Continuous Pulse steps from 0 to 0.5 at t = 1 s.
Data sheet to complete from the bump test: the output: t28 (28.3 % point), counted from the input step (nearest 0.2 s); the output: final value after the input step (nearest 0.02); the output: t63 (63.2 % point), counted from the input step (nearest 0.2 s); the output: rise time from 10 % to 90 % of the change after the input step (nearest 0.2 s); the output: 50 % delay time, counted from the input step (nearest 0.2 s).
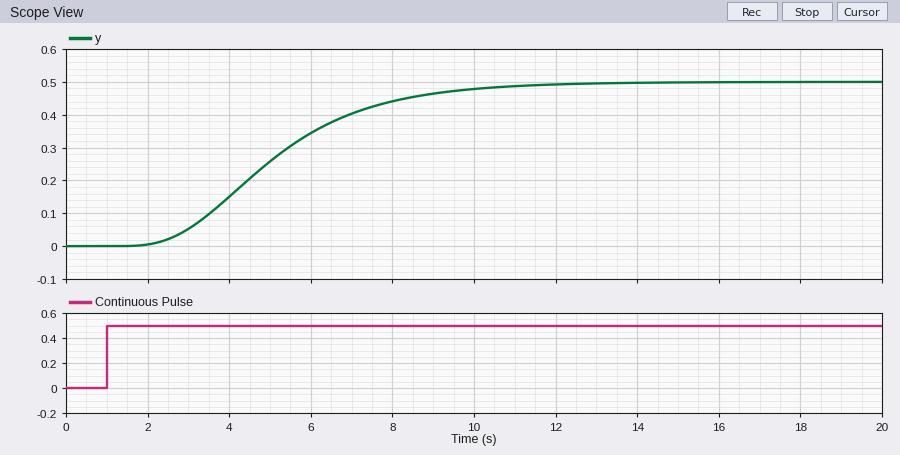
3.0 s
0.50
4.6 s
5.4 s
4.0 s
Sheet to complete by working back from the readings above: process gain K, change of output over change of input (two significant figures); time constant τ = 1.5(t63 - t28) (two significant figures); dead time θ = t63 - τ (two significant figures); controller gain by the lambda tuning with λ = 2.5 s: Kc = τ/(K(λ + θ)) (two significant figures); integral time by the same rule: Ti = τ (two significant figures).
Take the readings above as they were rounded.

1.0
2.4 s
2.2 s
0.51
2.4 s
